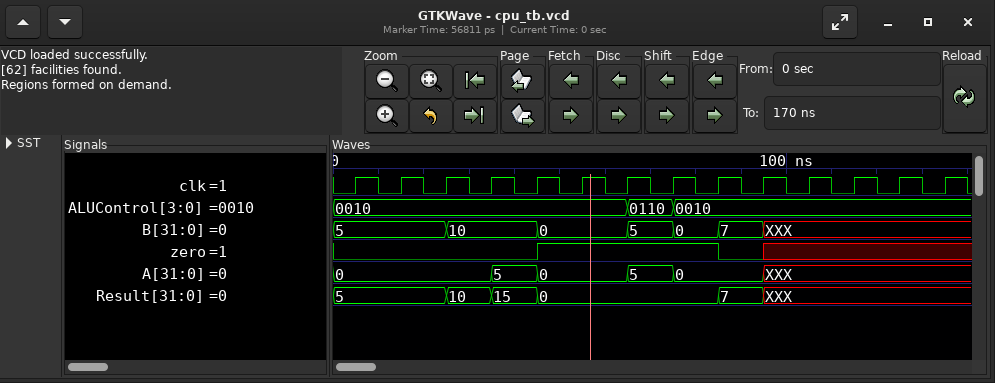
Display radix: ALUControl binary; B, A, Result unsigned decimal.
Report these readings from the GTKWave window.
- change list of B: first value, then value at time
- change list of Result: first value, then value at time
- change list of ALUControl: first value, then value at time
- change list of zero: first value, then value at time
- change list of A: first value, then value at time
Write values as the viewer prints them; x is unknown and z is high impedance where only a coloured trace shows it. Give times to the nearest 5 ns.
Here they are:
5, 10 at 25 ns, 0 at 45 ns, 5 at 65 ns, 0 at 75 ns, 7 at 85 ns, XXX at 95 ns
5, 10 at 25 ns, 15 at 35 ns, 0 at 45 ns, 7 at 85 ns, XXX at 95 ns
0010, 0110 at 65 ns, 0010 at 75 ns
0, 1 at 45 ns, 0 at 85 ns, x at 95 ns
0, 5 at 35 ns, 0 at 45 ns, 5 at 65 ns, 0 at 75 ns, XXX at 95 ns
